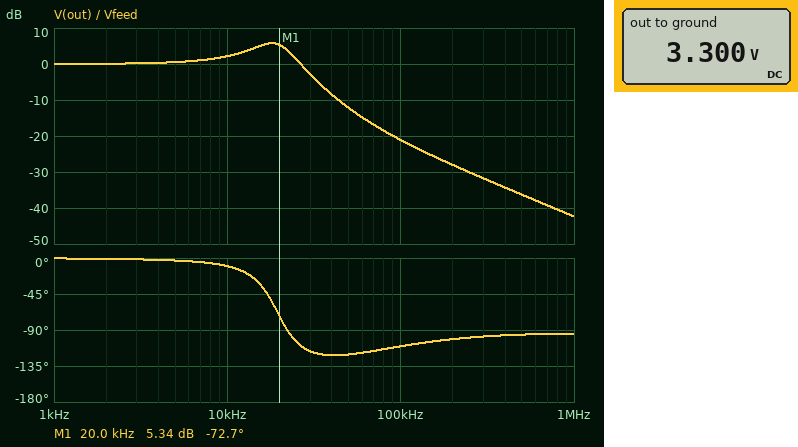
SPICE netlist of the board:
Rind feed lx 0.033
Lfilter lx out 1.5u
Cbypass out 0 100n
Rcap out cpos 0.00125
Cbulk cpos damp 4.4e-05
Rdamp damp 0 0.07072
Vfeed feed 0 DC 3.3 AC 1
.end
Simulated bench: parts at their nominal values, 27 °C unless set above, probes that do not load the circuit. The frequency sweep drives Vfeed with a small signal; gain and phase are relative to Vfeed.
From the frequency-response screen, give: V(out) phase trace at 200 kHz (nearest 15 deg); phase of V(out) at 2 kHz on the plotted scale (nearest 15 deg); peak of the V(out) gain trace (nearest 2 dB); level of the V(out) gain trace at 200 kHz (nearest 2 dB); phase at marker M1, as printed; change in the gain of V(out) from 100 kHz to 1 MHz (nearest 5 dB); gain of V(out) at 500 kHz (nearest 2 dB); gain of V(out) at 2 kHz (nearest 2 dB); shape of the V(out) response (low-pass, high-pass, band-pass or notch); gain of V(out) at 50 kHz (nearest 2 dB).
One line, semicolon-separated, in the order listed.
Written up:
-105 deg; 0 deg; 6 dB; -28 dB; -72.7 deg; -20 dB; -36 dB; 0 dB; low-pass; -12 dB
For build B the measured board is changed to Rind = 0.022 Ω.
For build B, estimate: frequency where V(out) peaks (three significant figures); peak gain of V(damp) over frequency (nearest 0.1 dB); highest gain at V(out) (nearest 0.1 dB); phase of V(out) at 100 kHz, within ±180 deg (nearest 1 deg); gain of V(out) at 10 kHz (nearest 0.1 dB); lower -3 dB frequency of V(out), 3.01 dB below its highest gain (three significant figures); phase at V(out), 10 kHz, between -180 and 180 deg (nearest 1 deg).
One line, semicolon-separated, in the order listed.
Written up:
18.4 kHz; -2.5 dB; 6.7 dB; -111 deg; 2.3 dB; 12.6 kHz; -8 deg
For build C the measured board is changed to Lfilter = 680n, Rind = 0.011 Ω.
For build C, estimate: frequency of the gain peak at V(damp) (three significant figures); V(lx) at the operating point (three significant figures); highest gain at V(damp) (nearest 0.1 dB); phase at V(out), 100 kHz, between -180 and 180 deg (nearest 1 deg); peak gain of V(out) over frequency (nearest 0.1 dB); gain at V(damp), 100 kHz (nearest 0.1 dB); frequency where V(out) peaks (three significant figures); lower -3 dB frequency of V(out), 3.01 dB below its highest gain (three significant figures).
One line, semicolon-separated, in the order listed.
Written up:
29.1 kHz; 3.30 V; -1.4 dB; -105 deg; 5.1 dB; -15.1 dB; 26.5 kHz; 14.5 kHz
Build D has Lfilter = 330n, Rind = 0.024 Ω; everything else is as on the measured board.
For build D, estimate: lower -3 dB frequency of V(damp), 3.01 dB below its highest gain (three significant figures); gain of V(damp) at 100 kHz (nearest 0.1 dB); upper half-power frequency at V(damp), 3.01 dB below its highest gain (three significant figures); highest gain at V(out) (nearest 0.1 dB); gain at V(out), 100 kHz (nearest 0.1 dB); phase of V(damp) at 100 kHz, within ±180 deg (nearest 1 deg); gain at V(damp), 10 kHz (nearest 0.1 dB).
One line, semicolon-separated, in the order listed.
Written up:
24.6 kHz; -8.9 dB; 70.8 kHz; 2.0 dB; -7.7 dB; -61 deg; -14.0 dB
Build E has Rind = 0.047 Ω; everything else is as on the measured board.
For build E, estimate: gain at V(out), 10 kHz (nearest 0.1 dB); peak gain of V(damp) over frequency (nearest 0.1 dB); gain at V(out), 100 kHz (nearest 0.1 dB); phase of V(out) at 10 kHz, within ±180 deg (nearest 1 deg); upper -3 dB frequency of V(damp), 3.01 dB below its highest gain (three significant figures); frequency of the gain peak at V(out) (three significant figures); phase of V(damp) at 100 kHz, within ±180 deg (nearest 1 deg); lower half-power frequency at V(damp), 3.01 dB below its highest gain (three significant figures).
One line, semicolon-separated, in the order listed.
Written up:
2.0 dB; -4.5 dB; -21.1 dB; -13 deg; 26.9 kHz; 17.7 kHz; -83 deg; 14.3 kHz
